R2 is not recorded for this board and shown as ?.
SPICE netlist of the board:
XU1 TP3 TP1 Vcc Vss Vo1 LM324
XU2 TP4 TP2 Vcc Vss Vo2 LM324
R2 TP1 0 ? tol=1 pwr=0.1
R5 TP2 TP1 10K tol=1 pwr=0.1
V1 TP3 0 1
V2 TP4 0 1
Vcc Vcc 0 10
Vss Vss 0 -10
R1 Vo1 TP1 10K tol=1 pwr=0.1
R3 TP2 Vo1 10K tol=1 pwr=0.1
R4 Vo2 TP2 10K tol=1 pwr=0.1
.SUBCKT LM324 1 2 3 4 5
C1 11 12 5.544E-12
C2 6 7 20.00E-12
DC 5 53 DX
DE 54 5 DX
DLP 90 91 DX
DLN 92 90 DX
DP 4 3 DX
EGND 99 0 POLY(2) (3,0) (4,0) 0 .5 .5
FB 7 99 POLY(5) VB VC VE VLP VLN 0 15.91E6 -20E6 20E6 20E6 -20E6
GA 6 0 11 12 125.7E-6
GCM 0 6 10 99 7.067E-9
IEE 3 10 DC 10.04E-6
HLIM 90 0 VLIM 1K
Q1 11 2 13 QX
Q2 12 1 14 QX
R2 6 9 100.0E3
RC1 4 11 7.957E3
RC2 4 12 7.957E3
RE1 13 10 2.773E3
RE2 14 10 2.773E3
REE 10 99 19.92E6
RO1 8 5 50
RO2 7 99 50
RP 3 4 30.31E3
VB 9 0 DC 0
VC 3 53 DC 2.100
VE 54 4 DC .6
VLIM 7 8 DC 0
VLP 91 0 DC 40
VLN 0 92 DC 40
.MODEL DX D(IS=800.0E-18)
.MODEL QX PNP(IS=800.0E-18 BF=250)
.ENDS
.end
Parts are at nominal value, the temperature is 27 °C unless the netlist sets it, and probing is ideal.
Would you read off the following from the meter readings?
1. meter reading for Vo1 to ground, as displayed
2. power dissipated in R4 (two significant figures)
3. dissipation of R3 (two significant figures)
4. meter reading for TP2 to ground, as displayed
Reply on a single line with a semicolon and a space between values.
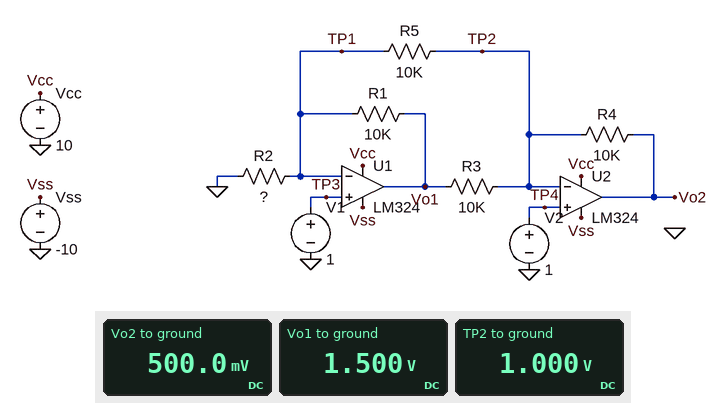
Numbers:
1.500 V; 25 µW; 25 µW; 1.000 V
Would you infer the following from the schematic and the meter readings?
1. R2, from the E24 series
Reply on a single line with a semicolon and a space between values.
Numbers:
20 kΩ
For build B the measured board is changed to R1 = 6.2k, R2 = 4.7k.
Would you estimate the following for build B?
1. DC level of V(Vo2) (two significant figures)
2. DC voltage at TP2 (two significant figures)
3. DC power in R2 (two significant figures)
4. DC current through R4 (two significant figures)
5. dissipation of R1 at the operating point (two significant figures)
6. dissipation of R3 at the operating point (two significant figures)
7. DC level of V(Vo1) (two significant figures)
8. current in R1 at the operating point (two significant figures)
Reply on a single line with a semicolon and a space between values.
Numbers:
-320 mV; 1.0 V; 210 µW; 130 µA; 280 µW; 170 µW; 2.3 V; 210 µA
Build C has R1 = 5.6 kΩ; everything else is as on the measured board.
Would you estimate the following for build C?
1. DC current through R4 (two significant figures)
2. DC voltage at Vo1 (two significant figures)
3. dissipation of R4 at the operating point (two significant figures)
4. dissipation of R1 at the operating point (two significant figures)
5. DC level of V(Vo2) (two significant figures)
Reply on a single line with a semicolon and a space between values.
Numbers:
28 µA; 1.3 V; 7.8 µW; 14 µW; 720 mV
